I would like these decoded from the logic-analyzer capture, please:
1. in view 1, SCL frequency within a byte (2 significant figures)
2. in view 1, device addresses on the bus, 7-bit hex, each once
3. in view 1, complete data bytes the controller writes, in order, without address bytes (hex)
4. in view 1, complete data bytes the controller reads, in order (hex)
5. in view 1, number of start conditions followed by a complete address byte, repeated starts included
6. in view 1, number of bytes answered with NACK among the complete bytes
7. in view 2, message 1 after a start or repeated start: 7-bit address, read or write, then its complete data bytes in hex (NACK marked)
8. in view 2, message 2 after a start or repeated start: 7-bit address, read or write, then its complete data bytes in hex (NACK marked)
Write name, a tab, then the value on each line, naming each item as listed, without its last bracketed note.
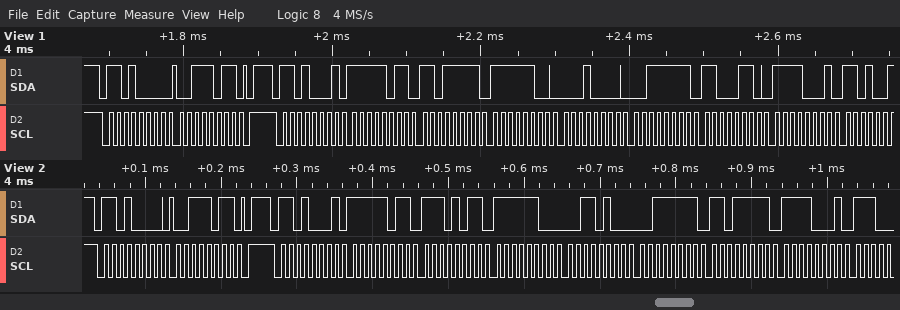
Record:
in view 1, SCL frequency within a byte	100 kHz
in view 1, device addresses on the bus, 7-bit hex, each once	0x68
in view 1, complete data bytes the controller writes, in order, without address bytes	3B
in view 1, complete data bytes the controller reads, in order	FB DF FC 10 3F C6 F1
in view 1, number of start conditions followed by a complete address byte, repeated starts included	2
in view 1, number of bytes answered with NACK among the complete bytes	0
in view 2, message 1 after a start or repeated start: 7-bit address, read or write, then its complete data bytes in hex	0x68 write: 3B
in view 2, message 2 after a start or repeated start: 7-bit address, read or write, then its complete data bytes in hex	0x68 read: FB EB FC 34 3F DF F1
